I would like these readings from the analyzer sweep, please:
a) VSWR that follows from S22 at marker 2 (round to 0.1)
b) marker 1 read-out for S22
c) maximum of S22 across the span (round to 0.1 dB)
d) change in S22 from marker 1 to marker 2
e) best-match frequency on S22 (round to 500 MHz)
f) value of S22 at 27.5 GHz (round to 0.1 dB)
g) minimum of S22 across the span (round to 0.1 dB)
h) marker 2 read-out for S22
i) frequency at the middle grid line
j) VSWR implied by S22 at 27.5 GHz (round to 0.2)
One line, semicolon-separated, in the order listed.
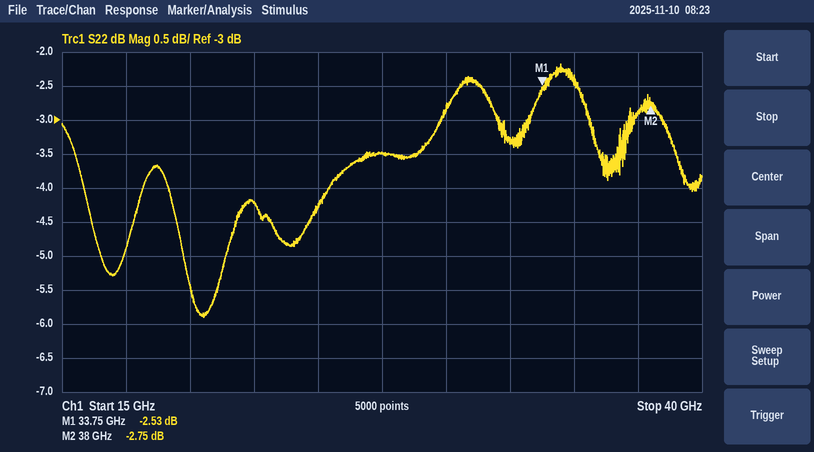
6.4; -2.53 dB; -2.2 dB; -0.22 dB; 20.5 GHz; -3.5 dB; -5.9 dB; -2.75 dB; 27.5 GHz; 5.0
